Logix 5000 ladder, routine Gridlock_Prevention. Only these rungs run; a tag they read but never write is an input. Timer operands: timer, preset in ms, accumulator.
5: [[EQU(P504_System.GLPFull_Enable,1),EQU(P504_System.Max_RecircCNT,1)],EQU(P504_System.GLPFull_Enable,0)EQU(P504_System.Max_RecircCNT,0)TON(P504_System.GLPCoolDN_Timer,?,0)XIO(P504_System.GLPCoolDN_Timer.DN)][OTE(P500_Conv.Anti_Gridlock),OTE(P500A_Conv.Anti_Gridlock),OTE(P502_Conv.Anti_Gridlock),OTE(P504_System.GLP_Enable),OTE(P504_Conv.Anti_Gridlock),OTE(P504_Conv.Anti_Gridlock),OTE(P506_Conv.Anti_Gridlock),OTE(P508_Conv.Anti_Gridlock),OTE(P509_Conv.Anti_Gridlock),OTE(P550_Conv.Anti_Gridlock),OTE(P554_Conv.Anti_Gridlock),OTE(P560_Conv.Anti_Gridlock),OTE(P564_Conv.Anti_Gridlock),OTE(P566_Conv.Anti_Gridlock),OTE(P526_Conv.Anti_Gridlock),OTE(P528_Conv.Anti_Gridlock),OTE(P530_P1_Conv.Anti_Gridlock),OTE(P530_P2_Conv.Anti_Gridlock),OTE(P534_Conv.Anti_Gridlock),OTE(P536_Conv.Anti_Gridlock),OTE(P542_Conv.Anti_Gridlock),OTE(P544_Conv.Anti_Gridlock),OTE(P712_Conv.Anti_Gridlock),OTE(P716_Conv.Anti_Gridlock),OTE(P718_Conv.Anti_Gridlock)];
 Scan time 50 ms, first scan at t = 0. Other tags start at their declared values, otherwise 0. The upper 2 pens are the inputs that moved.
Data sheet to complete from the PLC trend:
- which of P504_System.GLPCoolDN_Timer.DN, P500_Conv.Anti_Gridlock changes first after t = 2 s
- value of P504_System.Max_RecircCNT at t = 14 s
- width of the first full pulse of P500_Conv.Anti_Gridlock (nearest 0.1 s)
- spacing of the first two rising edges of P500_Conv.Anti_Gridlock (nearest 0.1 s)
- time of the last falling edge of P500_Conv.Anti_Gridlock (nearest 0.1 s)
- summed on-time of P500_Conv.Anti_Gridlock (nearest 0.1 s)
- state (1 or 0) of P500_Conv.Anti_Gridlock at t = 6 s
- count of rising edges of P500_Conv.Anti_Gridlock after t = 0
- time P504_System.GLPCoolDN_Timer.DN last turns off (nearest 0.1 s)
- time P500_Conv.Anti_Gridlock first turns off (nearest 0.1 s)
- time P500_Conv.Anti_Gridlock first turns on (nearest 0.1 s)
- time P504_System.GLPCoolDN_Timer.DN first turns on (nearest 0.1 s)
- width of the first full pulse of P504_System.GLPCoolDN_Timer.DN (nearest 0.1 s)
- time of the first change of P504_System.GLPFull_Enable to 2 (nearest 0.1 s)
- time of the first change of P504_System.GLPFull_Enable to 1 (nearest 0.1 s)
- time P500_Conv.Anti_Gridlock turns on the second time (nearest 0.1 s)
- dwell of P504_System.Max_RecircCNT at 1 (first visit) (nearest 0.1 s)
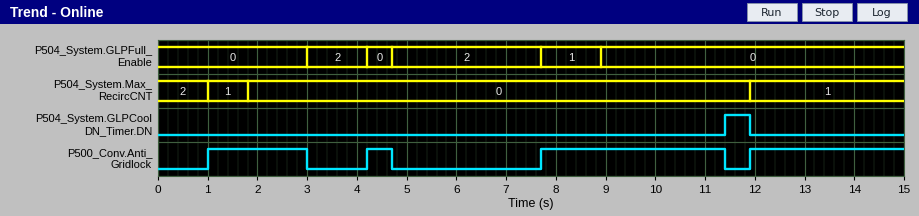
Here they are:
P500_Conv.Anti_Gridlock
1
2.0 s
3.2 s
11.4 s
9.3 s
0
4
11.9 s
3.0 s
1.0 s
11.4 s
0.5 s
3.0 s
7.7 s
4.2 s
0.8 s
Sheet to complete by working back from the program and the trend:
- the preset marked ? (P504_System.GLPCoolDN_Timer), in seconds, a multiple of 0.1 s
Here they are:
2.5 s
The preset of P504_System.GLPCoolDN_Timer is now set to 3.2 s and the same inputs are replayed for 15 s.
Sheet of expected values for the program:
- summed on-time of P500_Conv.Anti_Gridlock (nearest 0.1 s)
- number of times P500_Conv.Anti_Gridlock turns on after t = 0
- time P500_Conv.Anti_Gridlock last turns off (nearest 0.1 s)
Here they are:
9.8 s
3
4.7 s
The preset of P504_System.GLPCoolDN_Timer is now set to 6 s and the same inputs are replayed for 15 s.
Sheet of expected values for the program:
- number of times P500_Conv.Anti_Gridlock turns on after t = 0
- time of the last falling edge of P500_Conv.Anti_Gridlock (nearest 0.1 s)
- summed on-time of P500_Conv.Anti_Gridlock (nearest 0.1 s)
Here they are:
3
4.7 s
9.8 s
